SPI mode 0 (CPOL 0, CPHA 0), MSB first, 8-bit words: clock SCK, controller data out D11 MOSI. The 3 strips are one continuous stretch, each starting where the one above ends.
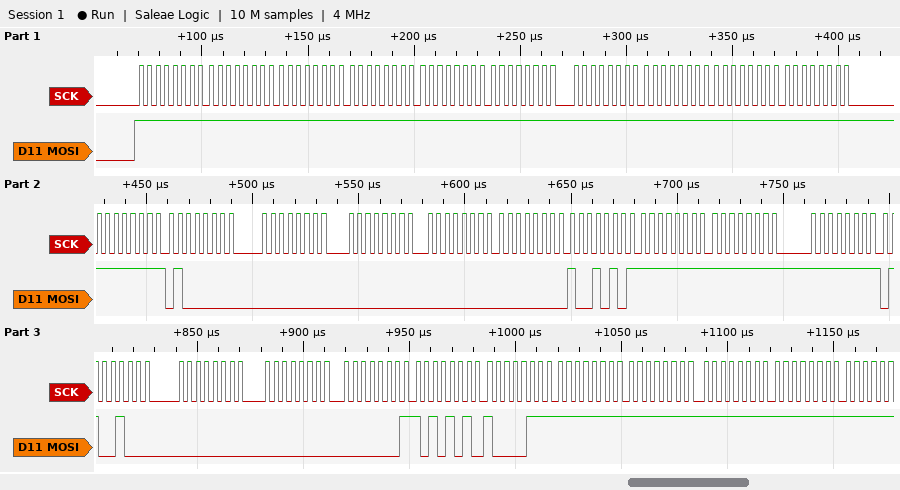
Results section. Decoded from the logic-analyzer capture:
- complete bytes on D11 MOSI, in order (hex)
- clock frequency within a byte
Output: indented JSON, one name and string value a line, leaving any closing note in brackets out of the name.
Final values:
{
  "complete bytes on D11 MOSI, in order": "FF FF FF FF FF FF FF FF FF FF FF 40 00 00 00 00 95 FF FF FF 48 00 00 01 AA 87 FF FF FF FF",
  "clock frequency within a byte": "250 kHz"
}
